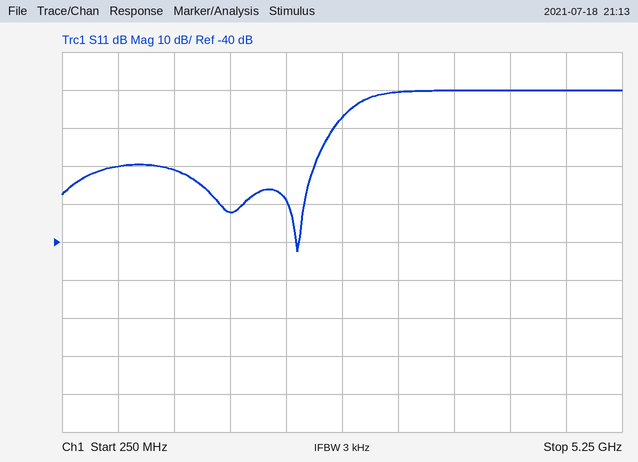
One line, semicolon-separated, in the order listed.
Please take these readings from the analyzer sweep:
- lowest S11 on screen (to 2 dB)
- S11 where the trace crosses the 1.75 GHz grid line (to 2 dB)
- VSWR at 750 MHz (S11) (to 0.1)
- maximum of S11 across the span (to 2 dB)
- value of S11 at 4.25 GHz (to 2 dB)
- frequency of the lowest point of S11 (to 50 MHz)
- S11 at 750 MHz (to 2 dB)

-42 dB; -32 dB; 1.2; 0 dB; 0 dB; 2.35 GHz; -20 dB
